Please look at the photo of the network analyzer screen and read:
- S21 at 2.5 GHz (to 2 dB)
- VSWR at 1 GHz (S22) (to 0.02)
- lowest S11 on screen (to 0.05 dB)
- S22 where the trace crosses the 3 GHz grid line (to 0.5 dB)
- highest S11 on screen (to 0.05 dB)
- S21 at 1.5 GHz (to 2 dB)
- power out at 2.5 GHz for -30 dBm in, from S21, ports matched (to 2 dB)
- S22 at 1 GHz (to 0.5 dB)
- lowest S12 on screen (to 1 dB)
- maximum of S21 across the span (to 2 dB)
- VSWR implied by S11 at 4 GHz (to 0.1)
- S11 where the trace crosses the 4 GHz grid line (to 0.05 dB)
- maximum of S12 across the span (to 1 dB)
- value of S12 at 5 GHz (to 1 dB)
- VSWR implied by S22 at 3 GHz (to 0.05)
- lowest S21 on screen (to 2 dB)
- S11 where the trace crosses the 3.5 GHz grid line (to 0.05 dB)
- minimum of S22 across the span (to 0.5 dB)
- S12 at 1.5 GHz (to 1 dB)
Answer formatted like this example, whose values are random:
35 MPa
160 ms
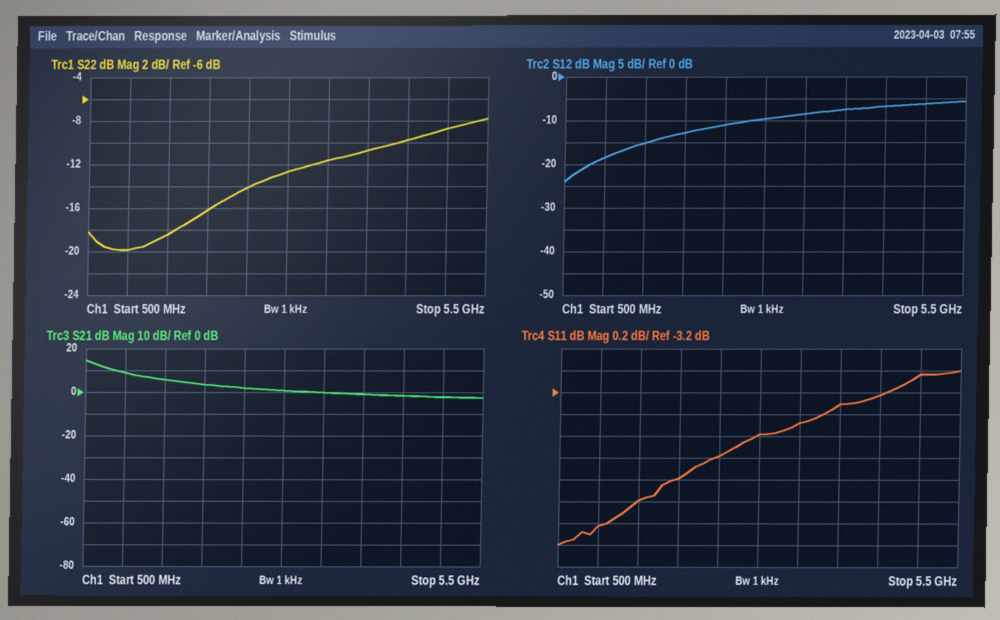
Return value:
2 dB
1.22
-4.60 dB
-12.5 dB
-3.00 dB
6 dB
-28 dBm
-20.0 dB
-24 dB
14 dB
5.3
-3.30 dB
-6 dB
-6 dB
1.60
-2 dB
-3.50 dB
-20.0 dB
-15 dB
